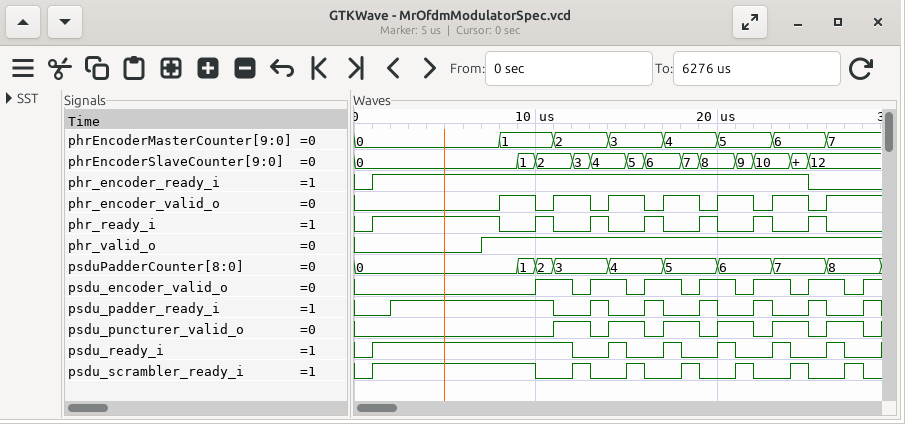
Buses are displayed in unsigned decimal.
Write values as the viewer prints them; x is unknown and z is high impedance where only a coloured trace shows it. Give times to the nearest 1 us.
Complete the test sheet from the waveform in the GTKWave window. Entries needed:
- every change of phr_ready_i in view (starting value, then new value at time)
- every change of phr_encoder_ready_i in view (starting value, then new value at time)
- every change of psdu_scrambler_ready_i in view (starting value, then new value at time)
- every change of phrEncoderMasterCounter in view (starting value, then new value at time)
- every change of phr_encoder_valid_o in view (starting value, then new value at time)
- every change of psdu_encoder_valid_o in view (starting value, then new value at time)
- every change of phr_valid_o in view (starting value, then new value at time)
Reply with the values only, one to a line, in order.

0, 1 at 1 us, 0 at 8 us, 1 at 10 us, 0 at 11 us, 1 at 13 us, 0 at 14 us, 1 at 16 us, 0 at 17 us, 1 at 19 us, 0 at 20 us, 1 at 22 us, 0 at 23 us, 1 at 25 us, 0 at 26 us
0, 1 at 1 us, 0 at 25 us
0, 1 at 1 us, 0 at 10 us, 1 at 12 us, 0 at 13 us, 1 at 15 us, 0 at 16 us, 1 at 18 us, 0 at 19 us, 1 at 21 us, 0 at 22 us, 1 at 24 us, 0 at 25 us, 1 at 27 us, 0 at 28 us
0, 1 at 8 us, 2 at 11 us, 3 at 14 us, 4 at 17 us, 5 at 20 us, 6 at 23 us, 7 at 26 us
0, 1 at 8 us, 0 at 10 us, 1 at 11 us, 0 at 13 us, 1 at 14 us, 0 at 16 us, 1 at 17 us, 0 at 19 us, 1 at 20 us, 0 at 22 us, 1 at 23 us, 0 at 25 us, 1 at 26 us
0, 1 at 10 us, 0 at 12 us, 1 at 13 us, 0 at 15 us, 1 at 16 us, 0 at 18 us, 1 at 19 us, 0 at 21 us, 1 at 22 us, 0 at 24 us, 1 at 25 us, 0 at 27 us, 1 at 28 us
0, 1 at 7 us
